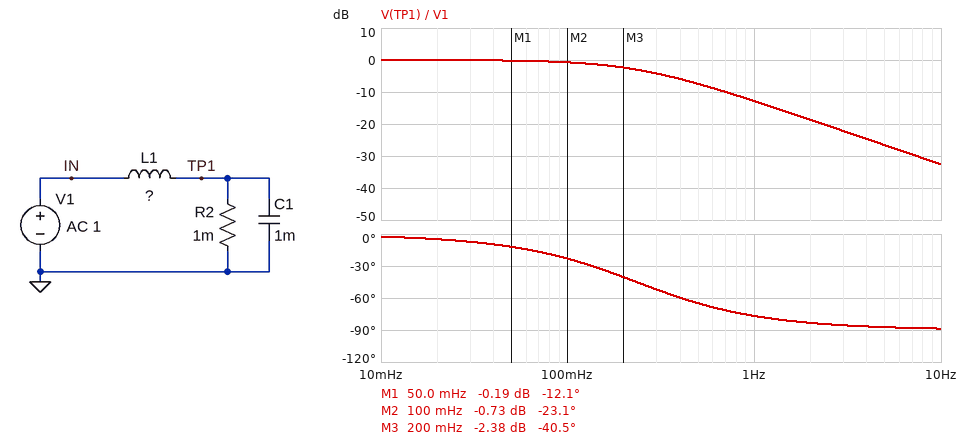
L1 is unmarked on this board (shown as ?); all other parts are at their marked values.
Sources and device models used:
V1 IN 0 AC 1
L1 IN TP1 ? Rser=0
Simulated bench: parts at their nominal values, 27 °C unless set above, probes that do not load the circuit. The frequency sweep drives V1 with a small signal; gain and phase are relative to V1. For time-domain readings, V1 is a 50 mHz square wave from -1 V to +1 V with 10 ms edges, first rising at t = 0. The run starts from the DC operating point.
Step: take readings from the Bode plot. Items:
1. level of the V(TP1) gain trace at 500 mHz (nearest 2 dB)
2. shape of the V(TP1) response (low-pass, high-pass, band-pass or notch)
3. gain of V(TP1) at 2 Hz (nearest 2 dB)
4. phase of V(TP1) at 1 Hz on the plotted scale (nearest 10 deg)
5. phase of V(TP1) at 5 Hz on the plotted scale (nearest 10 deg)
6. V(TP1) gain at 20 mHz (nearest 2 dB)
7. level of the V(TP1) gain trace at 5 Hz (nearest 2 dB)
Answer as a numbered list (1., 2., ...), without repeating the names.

1. -8 dB
2. low-pass
3. -18 dB
4. -80 deg
5. -90 deg
6. 0 dB
7. -26 dB
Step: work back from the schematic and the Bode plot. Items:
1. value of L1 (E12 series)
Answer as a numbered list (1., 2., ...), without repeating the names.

1. 680 µH
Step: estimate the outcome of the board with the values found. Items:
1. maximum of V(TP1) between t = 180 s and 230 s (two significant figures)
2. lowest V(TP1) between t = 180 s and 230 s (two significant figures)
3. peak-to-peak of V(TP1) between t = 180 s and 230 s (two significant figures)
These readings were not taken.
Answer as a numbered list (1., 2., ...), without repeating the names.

1. 1.0 V
2. -1.0 V
3. 2.0 V
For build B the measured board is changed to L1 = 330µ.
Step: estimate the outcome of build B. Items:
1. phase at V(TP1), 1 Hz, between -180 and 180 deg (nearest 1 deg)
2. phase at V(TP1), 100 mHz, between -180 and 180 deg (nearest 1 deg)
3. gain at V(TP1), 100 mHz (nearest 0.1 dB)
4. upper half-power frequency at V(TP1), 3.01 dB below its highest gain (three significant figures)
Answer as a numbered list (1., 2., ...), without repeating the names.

1. -64 deg
2. -12 deg
3. -0.2 dB
4. 482 mHz
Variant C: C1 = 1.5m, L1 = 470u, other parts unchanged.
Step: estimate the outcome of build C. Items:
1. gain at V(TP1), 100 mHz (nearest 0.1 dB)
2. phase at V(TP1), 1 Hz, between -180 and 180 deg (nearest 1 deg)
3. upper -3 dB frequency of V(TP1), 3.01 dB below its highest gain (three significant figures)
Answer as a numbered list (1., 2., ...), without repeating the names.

1. -0.4 dB
2. -71 deg
3. 339 mHz
